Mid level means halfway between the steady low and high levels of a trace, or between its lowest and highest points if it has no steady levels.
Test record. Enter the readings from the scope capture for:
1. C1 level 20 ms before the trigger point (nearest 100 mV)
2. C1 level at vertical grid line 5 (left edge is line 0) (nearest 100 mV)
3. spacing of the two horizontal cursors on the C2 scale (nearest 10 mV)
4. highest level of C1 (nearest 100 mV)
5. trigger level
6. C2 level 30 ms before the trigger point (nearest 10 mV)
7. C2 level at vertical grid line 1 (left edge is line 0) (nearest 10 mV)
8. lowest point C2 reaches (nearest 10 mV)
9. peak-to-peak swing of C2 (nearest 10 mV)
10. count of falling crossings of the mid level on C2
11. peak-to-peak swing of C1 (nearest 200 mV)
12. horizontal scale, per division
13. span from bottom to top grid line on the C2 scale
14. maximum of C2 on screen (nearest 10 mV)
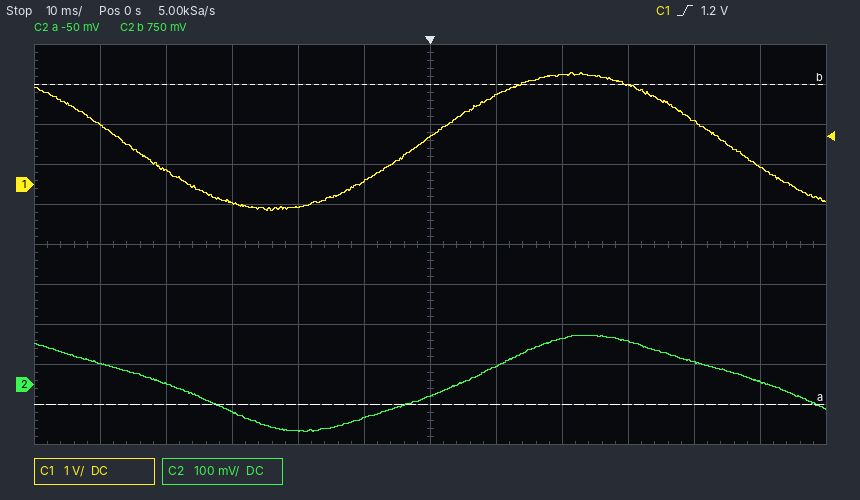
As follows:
-600 mV
100 mV
800 mV
2.8 V
1.2 V
-70 mV
50 mV
-120 mV
240 mV
2
3.4 V
10 ms
1 V
120 mV
